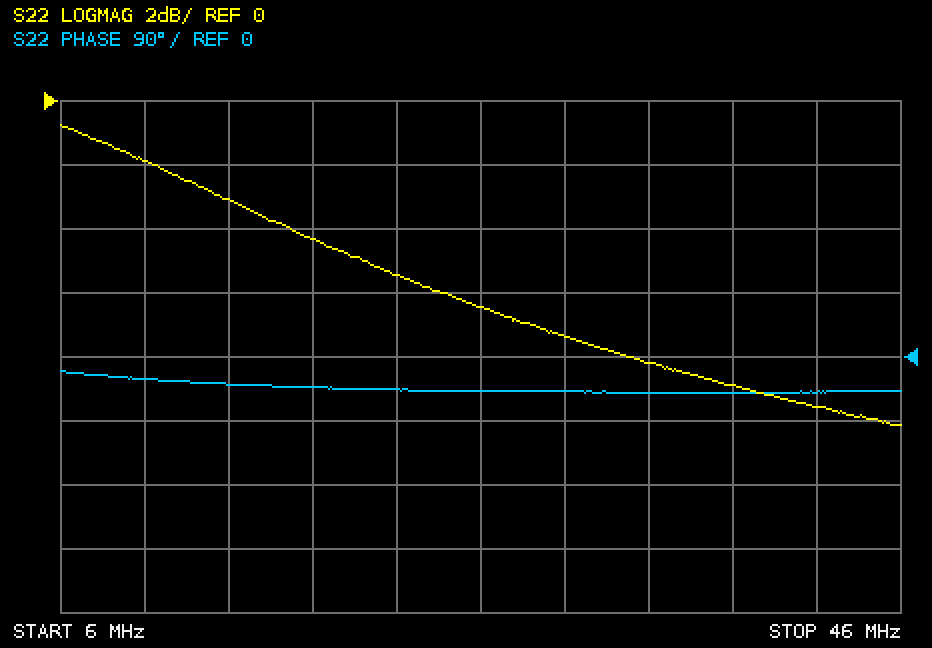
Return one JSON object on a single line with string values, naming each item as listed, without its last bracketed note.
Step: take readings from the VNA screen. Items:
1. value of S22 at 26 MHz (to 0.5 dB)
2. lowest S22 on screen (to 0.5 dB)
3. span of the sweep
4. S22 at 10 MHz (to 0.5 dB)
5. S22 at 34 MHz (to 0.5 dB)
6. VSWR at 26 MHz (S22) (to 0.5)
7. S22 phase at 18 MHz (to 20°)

{"value of S22 at 26 MHz": "-6.5 dB", "lowest S22 on screen": "-10.0 dB", "span of the sweep": "40 MHz", "S22 at 10 MHz": "-2.0 dB", "S22 at 34 MHz": "-8.0 dB", "VSWR at 26 MHz (S22)": "3.0", "S22 phase at 18 MHz": "-40°"}
